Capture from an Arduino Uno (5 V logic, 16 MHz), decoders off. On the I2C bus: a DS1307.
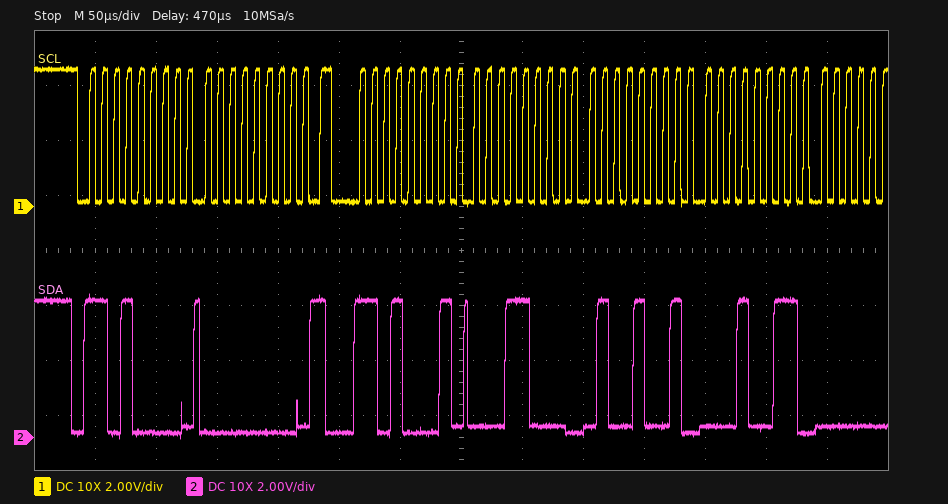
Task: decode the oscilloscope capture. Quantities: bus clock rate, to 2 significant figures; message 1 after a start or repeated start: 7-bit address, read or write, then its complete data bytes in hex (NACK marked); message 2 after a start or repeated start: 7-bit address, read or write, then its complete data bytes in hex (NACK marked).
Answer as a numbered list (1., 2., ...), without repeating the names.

1. 100 kHz
2. 0x68 write: 00
3. 0x68 read: 18 49 13
